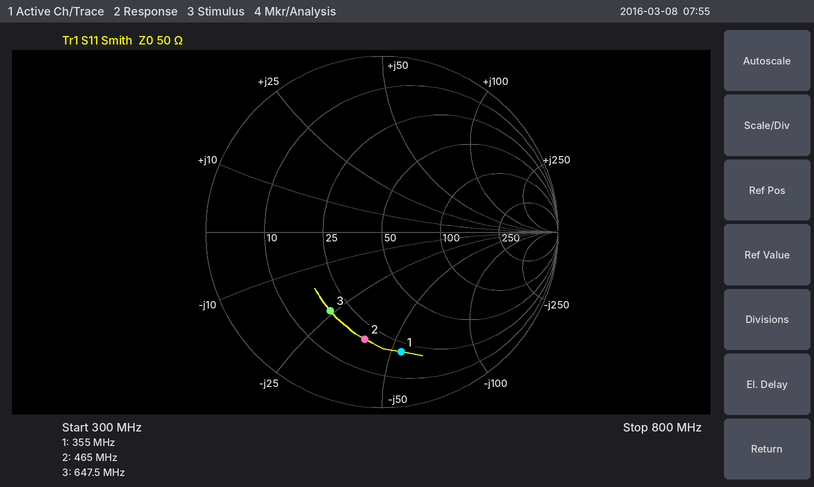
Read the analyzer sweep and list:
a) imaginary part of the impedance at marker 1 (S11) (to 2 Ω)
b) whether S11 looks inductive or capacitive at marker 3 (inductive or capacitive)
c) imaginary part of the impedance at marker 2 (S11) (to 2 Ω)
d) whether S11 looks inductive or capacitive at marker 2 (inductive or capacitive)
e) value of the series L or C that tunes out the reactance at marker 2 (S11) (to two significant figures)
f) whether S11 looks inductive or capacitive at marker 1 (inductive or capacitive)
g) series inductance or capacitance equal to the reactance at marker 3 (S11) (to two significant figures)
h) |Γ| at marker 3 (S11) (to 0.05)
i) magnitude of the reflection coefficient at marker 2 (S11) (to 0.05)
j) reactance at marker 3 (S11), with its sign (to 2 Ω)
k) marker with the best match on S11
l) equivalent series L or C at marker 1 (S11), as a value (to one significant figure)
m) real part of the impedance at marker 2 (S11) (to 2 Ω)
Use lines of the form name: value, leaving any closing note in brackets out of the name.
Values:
imaginary part of the impedance at marker 1 (S11): -54 Ω
whether S11 looks inductive or capacitive at marker 3: capacitive
imaginary part of the impedance at marker 2 (S11): -38 Ω
whether S11 looks inductive or capacitive at marker 2: capacitive
value of the series L or C that tunes out the reactance at marker 2 (S11): 13 nH
whether S11 looks inductive or capacitive at marker 1: capacitive
series inductance or capacitance equal to the reactance at marker 3 (S11): 10 pF
|Γ| at marker 3 (S11): 0.55
magnitude of the reflection coefficient at marker 2 (S11): 0.60
reactance at marker 3 (S11), with its sign: -24 Ω
marker with the best match on S11: marker 3
equivalent series L or C at marker 1 (S11), as a value: 8 pF
real part of the impedance at marker 2 (S11): 20 Ω
